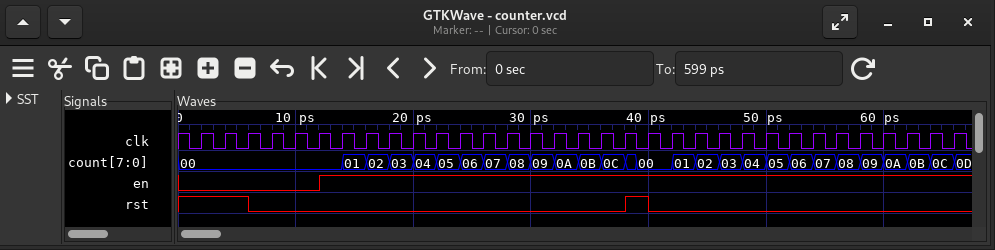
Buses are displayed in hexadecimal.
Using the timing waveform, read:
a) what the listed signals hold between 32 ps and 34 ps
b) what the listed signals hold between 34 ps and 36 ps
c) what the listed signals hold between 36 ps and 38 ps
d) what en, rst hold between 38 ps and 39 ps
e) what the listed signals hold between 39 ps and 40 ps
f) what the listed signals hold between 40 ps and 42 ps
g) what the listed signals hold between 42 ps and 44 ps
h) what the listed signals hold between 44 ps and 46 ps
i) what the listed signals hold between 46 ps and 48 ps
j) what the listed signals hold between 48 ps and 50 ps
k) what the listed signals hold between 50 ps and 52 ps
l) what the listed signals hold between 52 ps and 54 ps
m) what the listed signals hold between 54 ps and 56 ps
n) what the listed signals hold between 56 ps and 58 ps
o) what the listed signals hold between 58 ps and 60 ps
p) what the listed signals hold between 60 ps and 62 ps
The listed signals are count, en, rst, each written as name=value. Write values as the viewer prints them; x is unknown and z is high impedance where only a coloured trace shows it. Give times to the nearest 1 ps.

count=0A, en=1, rst=0
count=0B, en=1, rst=0
count=0C, en=1, rst=0
en=1, rst=1
count=00, en=1, rst=1
count=00, en=1, rst=0
count=01, en=1, rst=0
count=02, en=1, rst=0
count=03, en=1, rst=0
count=04, en=1, rst=0
count=05, en=1, rst=0
count=06, en=1, rst=0
count=07, en=1, rst=0
count=08, en=1, rst=0
count=09, en=1, rst=0
count=0A, en=1, rst=0
